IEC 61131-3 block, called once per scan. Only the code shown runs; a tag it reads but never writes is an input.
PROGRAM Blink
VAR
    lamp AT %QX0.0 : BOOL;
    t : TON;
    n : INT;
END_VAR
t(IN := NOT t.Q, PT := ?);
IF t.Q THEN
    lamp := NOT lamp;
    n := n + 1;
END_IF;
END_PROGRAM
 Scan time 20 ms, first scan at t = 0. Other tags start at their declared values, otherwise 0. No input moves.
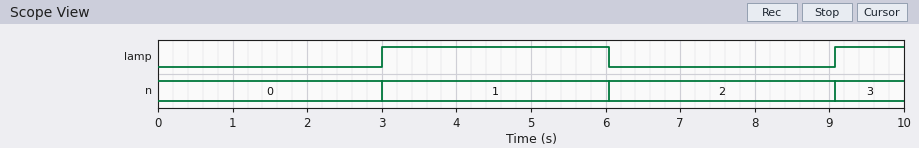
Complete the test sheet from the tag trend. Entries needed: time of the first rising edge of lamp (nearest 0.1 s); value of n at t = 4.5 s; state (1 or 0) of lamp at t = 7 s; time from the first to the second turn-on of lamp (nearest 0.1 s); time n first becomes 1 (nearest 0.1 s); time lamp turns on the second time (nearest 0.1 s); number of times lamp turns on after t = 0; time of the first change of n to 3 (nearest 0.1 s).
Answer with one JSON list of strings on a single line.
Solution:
["3.0 s", "1", "0", "6.1 s", "3.0 s", "9.1 s", "2", "9.1 s"]
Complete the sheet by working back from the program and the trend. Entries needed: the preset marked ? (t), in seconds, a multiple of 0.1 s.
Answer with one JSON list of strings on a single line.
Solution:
["3.0 s"]
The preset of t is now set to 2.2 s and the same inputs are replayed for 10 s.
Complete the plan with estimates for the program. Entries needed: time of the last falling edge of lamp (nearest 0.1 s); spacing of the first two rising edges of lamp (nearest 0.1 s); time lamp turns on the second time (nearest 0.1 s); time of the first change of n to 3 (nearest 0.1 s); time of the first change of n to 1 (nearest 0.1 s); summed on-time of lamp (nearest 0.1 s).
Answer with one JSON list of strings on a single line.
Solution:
["8.9 s", "4.5 s", "6.7 s", "6.7 s", "2.2 s", "4.5 s"]
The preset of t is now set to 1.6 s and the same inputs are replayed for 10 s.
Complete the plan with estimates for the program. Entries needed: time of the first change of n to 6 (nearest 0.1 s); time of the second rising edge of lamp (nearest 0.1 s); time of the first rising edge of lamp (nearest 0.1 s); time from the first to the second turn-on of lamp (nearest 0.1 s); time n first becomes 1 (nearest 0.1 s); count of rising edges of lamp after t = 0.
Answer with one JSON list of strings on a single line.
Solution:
["9.8 s", "4.9 s", "1.6 s", "3.3 s", "1.6 s", "3"]
